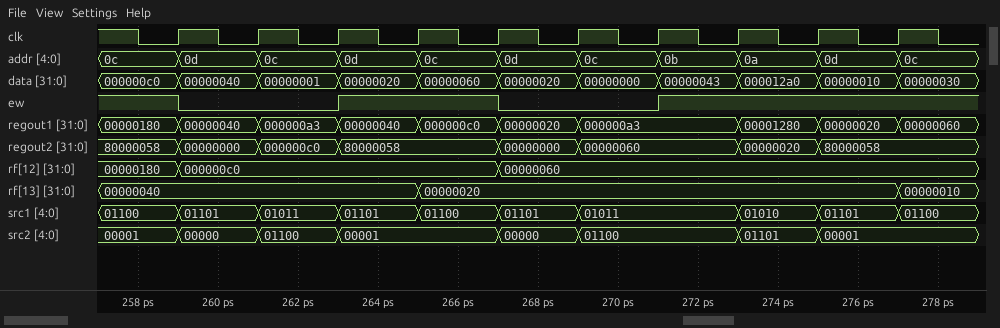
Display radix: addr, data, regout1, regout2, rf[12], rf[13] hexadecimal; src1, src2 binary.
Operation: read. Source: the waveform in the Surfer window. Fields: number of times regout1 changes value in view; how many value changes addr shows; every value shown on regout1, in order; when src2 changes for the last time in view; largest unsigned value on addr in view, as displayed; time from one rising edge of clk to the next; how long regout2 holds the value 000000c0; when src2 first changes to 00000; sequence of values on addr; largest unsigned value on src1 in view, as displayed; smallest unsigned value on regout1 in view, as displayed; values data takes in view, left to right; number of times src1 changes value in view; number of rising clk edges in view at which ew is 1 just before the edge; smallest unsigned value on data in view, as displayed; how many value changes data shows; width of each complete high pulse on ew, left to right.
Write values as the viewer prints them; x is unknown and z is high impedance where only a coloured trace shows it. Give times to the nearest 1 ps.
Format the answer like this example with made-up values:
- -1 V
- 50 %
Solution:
- 9
- 10
- 00000180, 00000040, 000000a3, 00000040, 000000c0, 00000020, 000000a3, 00001280, 00000020, 00000060
- 275 ps
- 0d
- 2 ps
- 2 ps
- 259 ps
- 0c, 0d, 0c, 0d, 0c, 0d, 0c, 0b, 0a, 0d, 0c
- 01101
- 00000020
- 000000c0, 00000040, 00000001, 00000020, 00000060, 00000020, 00000000, 00000043, 000012a0, 00000010, 00000030
- 9
- 6
- 00000000
- 10
- 4 ps
